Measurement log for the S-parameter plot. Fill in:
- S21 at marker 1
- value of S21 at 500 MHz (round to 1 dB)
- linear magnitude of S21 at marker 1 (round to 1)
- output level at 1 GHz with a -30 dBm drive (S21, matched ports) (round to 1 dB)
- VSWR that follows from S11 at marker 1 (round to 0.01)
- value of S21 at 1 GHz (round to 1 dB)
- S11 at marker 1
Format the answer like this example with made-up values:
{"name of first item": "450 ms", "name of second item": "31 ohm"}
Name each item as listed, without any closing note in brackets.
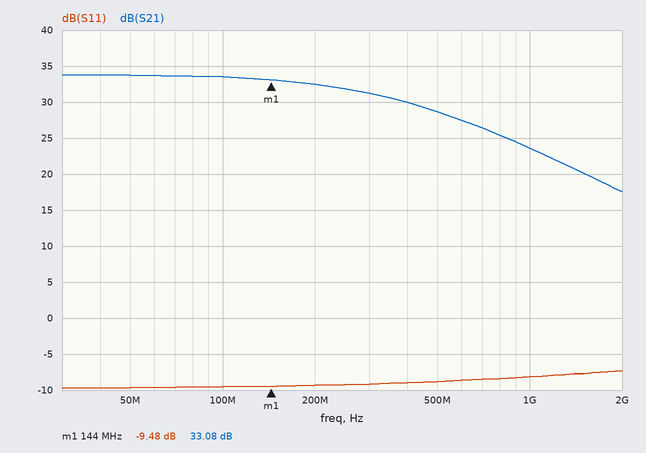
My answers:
{"S21 at marker 1": "33.08 dB", "value of S21 at 500 MHz": "29 dB", "linear magnitude of S21 at marker 1": "45", "output level at 1 GHz with a -30 dBm drive (S21, matched ports)": "-6 dBm", "VSWR that follows from S11 at marker 1": "2.01", "value of S21 at 1 GHz": "24 dB", "S11 at marker 1": "-9.48 dB"}
